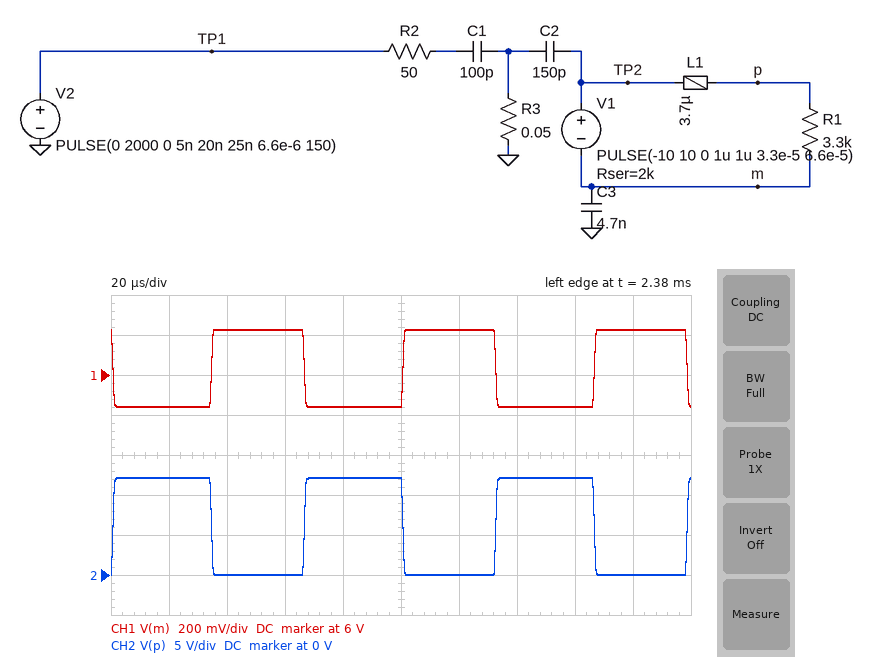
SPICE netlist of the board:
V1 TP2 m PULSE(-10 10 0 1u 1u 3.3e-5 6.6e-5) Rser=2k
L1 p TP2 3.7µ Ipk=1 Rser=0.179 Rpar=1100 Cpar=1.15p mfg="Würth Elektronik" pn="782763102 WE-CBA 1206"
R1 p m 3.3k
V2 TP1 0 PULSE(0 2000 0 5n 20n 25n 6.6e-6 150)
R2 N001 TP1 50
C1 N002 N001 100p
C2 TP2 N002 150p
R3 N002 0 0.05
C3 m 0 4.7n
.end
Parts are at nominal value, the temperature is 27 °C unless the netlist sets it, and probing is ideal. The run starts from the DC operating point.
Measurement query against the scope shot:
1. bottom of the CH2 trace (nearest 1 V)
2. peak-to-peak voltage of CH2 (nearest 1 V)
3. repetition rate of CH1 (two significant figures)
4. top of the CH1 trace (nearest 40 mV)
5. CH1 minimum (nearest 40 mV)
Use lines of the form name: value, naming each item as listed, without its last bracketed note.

bottom of the CH2 trace: 0 V
peak-to-peak voltage of CH2: 12 V
repetition rate of CH1: 15 kHz
top of the CH1 trace: 6.24 V
CH1 minimum: 5.84 V
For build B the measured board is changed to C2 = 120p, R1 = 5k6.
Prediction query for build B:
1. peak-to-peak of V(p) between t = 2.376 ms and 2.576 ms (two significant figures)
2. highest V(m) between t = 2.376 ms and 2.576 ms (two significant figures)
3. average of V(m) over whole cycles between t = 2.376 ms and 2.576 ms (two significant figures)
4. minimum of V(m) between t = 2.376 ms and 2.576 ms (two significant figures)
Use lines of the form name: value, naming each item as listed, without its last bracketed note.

peak-to-peak of V(p) between t = 2.376 ms and 2.576 ms: 14 V
highest V(m) between t = 2.376 ms and 2.576 ms: 7.4 V
average of V(m) over whole cycles between t = 2.376 ms and 2.576 ms: 7.2 V
minimum of V(m) between t = 2.376 ms and 2.576 ms: 7.0 V
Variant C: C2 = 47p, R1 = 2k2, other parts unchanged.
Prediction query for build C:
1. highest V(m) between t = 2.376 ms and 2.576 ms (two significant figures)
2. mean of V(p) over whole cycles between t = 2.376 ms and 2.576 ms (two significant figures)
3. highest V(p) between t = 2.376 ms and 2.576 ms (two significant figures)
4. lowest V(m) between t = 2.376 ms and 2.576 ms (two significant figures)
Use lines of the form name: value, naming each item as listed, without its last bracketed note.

highest V(m) between t = 2.376 ms and 2.576 ms: 5.2 V
mean of V(p) over whole cycles between t = 2.376 ms and 2.576 ms: 5.3 V
highest V(p) between t = 2.376 ms and 2.576 ms: 10 V
lowest V(m) between t = 2.376 ms and 2.576 ms: 5.1 V
